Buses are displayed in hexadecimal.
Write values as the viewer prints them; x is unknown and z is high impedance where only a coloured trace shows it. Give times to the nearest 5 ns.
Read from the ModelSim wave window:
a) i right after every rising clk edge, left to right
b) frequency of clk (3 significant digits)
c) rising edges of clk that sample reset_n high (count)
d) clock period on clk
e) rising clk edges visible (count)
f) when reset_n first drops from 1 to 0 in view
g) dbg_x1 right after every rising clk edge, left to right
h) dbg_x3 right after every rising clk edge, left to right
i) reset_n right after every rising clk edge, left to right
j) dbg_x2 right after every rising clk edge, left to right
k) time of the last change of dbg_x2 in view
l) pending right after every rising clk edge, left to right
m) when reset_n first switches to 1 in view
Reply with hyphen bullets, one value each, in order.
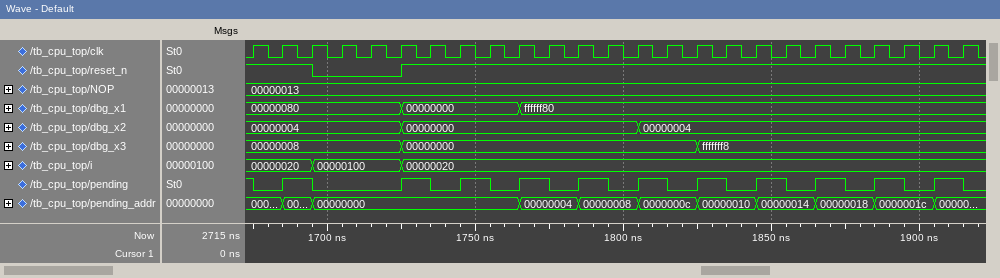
- 00000020, 00000020, 00000100, 00000100, 00000100, 00000020, 00000020, 00000020, 00000020, 00000020, 00000020, 00000020, 00000020, 00000020, 00000020, 00000020, 00000020, 00000020, 00000020, 00000020, 00000020, 00000020, 00000020, 00000020, 00000020
- 100 MHz
- 22
- 10 ns
- 25
- 1695 ns
- 00000080, 00000080, 00000080, 00000080, 00000080, 00000000, 00000000, 00000000, 00000000, ffffff80, ffffff80, ffffff80, ffffff80, ffffff80, ffffff80, ffffff80, ffffff80, ffffff80, ffffff80, ffffff80, ffffff80, ffffff80, ffffff80, ffffff80, ffffff80
- 00000008, 00000008, 00000008, 00000008, 00000008, 00000000, 00000000, 00000000, 00000000, 00000000, 00000000, 00000000, 00000000, 00000000, 00000000, fffffff8, fffffff8, fffffff8, fffffff8, fffffff8, fffffff8, fffffff8, fffffff8, fffffff8, fffffff8
- 1 1 0 0 0 1 1 1 1 1 1 1 1 1 1 1 1 1 1 1 1 1 1 1 1
- 00000004, 00000004, 00000004, 00000004, 00000004, 00000000, 00000000, 00000000, 00000000, 00000000, 00000000, 00000000, 00000000, 00000004, 00000004, 00000004, 00000004, 00000004, 00000004, 00000004, 00000004, 00000004, 00000004, 00000004, 00000004
- 1805 ns
- 0 1 0 0 0 1 0 1 0 1 0 1 0 1 0 1 0 1 0 1 0 1 0 1 0
- 1725 ns
